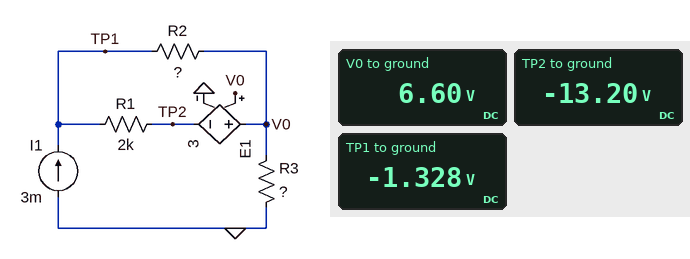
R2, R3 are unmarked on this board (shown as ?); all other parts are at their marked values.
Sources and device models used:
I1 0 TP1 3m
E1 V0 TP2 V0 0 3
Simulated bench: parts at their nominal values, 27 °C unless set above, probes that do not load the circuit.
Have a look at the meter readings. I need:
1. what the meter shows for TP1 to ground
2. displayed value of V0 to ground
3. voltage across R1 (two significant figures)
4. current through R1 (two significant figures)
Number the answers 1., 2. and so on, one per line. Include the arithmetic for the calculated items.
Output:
1. -1.328 V
2. 6.60 V
3. -1.328 V - (-13.2 V) = 12 V
4. (-1.328 V - (-13.2 V)) / 2 kΩ = 5.9 mA
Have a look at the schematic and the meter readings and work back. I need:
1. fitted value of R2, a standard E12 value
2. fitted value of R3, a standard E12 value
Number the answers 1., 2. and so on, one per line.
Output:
1. 2.7 kΩ
2. 2.2 kΩ
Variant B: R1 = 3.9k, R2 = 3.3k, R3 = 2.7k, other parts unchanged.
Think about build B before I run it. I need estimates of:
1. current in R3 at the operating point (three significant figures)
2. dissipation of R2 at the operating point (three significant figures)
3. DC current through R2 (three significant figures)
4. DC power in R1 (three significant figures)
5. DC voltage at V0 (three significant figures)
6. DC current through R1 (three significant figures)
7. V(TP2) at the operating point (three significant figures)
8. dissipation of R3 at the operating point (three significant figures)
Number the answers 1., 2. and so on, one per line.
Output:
1. 3.00 mA
2. 10.1 mW
3. 1.75 mA
4. 88.0 mW
5. 8.10 V
6. 4.75 mA
7. -16.2 V
8. 24.3 mW
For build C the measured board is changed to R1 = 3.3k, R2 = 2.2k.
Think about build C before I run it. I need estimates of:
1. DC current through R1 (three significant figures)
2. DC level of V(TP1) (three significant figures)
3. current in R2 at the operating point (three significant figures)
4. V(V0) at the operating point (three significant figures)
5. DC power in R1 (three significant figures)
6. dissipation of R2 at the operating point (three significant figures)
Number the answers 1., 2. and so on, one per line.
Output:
1. 4.80 mA
2. 2.64 V
3. 1.80 mA
4. 6.60 V
5. 76.0 mW
6. 7.13 mW
